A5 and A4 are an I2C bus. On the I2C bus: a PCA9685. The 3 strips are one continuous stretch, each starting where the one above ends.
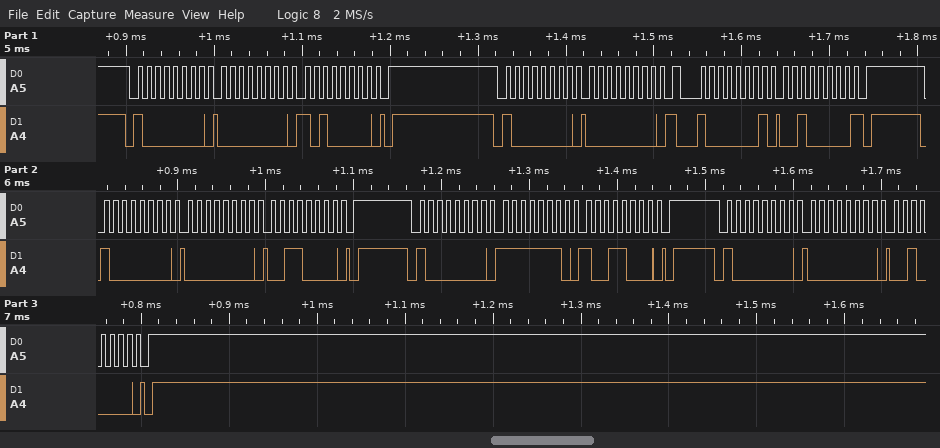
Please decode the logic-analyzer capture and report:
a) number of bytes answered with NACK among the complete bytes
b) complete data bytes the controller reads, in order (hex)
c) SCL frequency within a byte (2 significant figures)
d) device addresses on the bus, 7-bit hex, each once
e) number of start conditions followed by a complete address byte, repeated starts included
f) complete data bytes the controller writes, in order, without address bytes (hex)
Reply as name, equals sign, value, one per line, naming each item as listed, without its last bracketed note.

number of bytes answered with NACK among the complete bytes = 1
complete data bytes the controller reads, in order = 20
SCL frequency within a byte = 100 kHz
device addresses on the bus, 7-bit hex, each once = 0x40
number of start conditions followed by a complete address byte, repeated starts included = 6
complete data bytes the controller writes, in order, without address bytes = 00 A0 00 00 30 FE 98 00 20
